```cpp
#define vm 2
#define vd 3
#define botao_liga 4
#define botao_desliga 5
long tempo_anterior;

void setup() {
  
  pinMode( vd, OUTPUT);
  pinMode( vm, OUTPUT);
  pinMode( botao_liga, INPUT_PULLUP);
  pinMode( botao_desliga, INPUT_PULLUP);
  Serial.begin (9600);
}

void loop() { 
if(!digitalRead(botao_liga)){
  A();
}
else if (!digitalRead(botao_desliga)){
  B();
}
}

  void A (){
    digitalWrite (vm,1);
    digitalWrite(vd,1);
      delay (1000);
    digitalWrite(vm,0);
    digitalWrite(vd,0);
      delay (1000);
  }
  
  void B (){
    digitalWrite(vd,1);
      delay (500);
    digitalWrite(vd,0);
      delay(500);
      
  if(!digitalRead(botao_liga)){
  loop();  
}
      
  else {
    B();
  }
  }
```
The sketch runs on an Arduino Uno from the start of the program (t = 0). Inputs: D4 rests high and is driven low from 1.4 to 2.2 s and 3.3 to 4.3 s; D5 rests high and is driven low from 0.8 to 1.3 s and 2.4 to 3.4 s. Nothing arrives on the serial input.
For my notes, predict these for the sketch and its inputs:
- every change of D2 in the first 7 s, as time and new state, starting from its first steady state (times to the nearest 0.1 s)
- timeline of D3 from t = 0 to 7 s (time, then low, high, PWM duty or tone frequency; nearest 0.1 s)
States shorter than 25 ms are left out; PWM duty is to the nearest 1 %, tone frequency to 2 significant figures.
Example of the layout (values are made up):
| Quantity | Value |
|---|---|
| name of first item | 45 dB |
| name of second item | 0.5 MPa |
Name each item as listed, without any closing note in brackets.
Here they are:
| Quantity | Value |
|---|---|
| every change of D2 in the first 7 s, as time and new state, starting from its first steady state | 0 s low; 1.8 s high; 2.8 s low; 3.8 s high; 4.8 s low |
| timeline of D3 from t = 0 to 7 s | 0 s low; 0.8 s high; 1.3 s low; 1.8 s high; 2.8 s low; 3.8 s high; 4.8 s low |
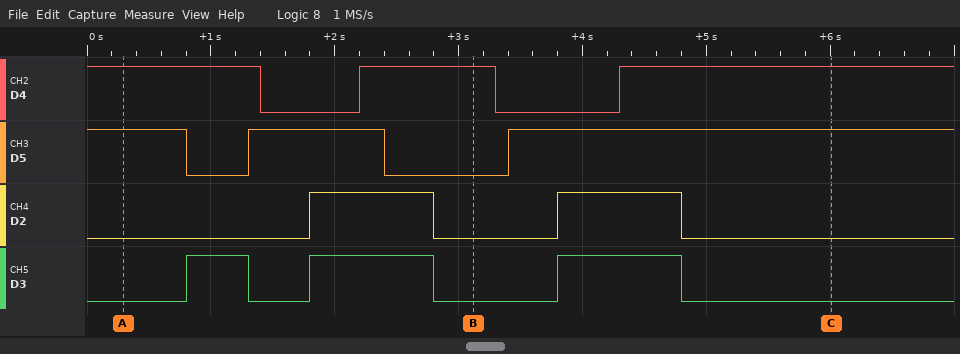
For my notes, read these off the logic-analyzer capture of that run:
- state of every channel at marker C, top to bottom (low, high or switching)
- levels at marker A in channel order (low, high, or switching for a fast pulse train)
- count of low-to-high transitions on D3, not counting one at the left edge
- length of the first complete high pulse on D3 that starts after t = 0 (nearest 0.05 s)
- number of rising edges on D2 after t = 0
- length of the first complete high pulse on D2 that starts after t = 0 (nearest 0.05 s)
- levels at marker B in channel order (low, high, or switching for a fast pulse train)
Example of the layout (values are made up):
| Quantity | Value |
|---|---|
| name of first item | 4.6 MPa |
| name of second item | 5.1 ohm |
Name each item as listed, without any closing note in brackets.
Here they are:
| Quantity | Value |
|---|---|
| state of every channel at marker C, top to bottom | D4 high, D5 high, D2 low, D3 low |
| levels at marker A in channel order | D4 high, D5 high, D2 low, D3 low |
| count of low-to-high transitions on D3, not counting one at the left edge | 3 |
| length of the first complete high pulse on D3 that starts after t = 0 | 0.50 s |
| number of rising edges on D2 after t = 0 | 2 |
| length of the first complete high pulse on D2 that starts after t = 0 | 1.00 s |
| levels at marker B in channel order | D4 high, D5 low, D2 low, D3 low |
